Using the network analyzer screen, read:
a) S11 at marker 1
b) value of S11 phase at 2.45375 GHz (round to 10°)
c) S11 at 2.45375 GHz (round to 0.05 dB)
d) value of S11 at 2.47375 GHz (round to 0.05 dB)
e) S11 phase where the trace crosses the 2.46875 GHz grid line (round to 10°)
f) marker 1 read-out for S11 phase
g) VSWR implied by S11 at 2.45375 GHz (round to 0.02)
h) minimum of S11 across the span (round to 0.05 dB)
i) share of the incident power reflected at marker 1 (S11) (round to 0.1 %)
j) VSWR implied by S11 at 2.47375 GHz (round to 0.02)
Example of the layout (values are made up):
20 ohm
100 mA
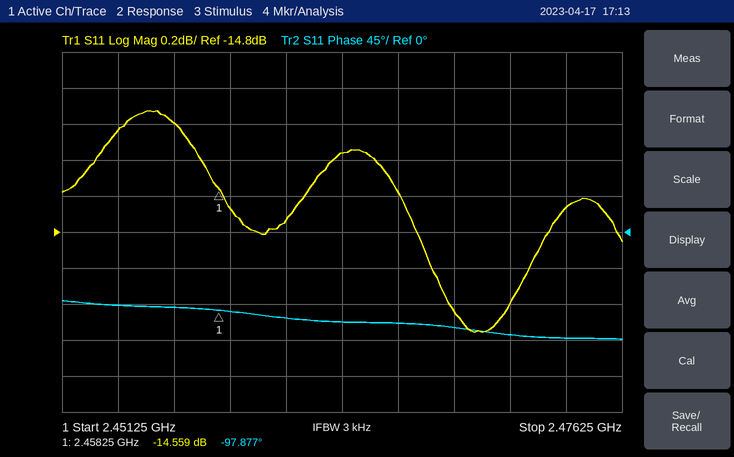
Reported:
-14.559 dB
-90°
-14.25 dB
-14.65 dB
-120°
-97.877°
1.48
-15.35 dB
3.5 %
1.46
